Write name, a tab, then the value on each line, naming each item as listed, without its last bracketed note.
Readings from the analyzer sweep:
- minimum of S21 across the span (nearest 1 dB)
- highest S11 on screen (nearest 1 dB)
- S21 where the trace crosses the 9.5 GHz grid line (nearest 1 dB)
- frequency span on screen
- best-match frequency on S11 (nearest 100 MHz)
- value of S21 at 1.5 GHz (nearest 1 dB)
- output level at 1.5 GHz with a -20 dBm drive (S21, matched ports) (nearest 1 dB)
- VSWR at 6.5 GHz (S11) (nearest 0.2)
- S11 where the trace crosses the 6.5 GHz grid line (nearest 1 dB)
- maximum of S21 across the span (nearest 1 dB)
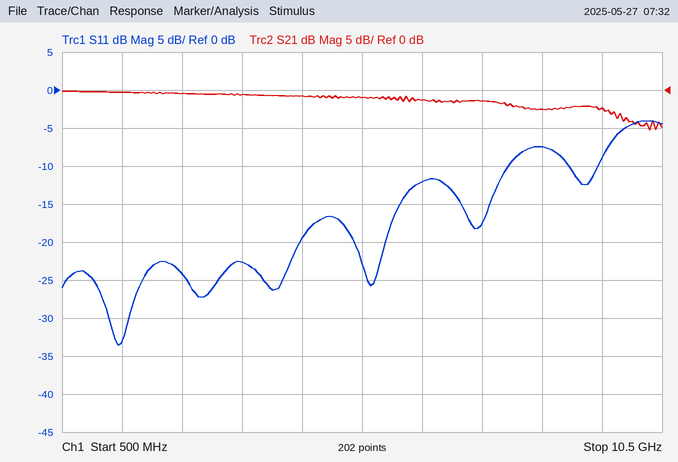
minimum of S21 across the span	-5 dB
highest S11 on screen	-4 dB
S21 where the trace crosses the 9.5 GHz grid line	-2 dB
frequency span on screen	10 GHz
best-match frequency on S11	1.4 GHz
value of S21 at 1.5 GHz	0 dB
output level at 1.5 GHz with a -20 dBm drive (S21, matched ports)	-20 dBm
VSWR at 6.5 GHz (S11)	1.6
S11 where the trace crosses the 6.5 GHz grid line	-12 dB
maximum of S21 across the span	0 dB
